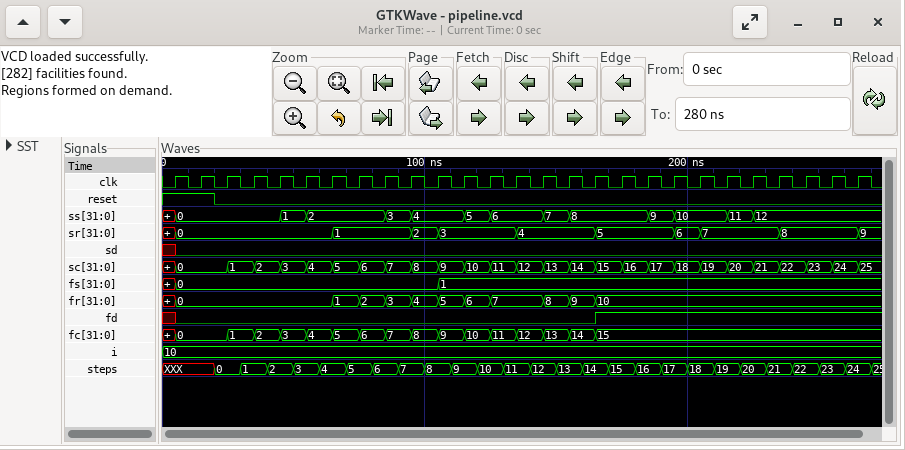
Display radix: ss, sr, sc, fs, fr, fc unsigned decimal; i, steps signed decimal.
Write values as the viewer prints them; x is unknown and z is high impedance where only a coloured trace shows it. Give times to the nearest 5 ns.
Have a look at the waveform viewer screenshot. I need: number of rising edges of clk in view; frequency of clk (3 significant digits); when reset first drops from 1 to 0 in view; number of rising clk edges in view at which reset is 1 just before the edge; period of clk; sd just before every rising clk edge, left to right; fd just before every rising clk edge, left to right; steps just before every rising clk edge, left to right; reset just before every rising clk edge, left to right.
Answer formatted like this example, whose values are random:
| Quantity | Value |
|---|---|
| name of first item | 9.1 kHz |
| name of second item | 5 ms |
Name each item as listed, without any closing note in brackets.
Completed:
| Quantity | Value |
|---|---|
| number of rising edges of clk in view | 27 |
| frequency of clk | 100 MHz |
| when reset first drops from 1 to 0 in view | 20 ns |
| number of rising clk edges in view at which reset is 1 just before the edge | 2 |
| period of clk | 10 ns |
| sd just before every rising clk edge, left to right | x 0 0 0 0 0 0 0 0 0 0 0 0 0 0 0 0 0 0 0 0 0 0 0 0 0 0 |
| fd just before every rising clk edge, left to right | x 0 0 0 0 0 0 0 0 0 0 0 0 0 0 0 0 1 1 1 1 1 1 1 1 1 1 |
| steps just before every rising clk edge, left to right | XXX, XXX, 0, 1, 2, 3, 4, 5, 6, 7, 8, 9, 10, 11, 12, 13, 14, 15, 16, 17, 18, 19, 20, 21, 22, 23, 24 |
| reset just before every rising clk edge, left to right | 1 1 0 0 0 0 0 0 0 0 0 0 0 0 0 0 0 0 0 0 0 0 0 0 0 0 0 |
